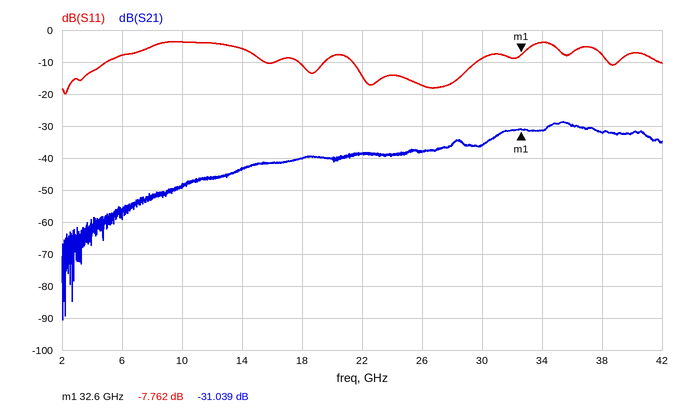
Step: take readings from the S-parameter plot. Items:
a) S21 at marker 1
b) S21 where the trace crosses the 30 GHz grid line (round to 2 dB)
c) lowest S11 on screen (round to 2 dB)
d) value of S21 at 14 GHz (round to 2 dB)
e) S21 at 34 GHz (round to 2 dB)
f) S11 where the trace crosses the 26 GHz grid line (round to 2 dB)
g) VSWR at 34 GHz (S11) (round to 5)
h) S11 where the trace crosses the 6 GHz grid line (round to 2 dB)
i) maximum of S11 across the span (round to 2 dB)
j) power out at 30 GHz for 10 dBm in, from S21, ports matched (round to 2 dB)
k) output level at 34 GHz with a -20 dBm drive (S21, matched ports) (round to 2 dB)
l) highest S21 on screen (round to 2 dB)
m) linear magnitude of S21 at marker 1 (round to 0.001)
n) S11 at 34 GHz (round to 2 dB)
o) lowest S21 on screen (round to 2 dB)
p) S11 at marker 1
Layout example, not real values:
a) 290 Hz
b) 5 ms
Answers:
a) -31.039 dB
b) -36 dB
c) -20 dB
d) -44 dB
e) -32 dB
f) -18 dB
g) 5
h) -8 dB
i) -4 dB
j) -26 dBm
k) -52 dBm
l) -28 dB
m) 0.028
n) -4 dB
o) -90 dB
p) -7.762 dB
